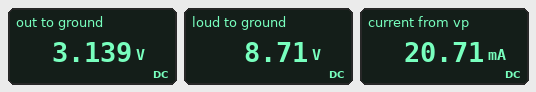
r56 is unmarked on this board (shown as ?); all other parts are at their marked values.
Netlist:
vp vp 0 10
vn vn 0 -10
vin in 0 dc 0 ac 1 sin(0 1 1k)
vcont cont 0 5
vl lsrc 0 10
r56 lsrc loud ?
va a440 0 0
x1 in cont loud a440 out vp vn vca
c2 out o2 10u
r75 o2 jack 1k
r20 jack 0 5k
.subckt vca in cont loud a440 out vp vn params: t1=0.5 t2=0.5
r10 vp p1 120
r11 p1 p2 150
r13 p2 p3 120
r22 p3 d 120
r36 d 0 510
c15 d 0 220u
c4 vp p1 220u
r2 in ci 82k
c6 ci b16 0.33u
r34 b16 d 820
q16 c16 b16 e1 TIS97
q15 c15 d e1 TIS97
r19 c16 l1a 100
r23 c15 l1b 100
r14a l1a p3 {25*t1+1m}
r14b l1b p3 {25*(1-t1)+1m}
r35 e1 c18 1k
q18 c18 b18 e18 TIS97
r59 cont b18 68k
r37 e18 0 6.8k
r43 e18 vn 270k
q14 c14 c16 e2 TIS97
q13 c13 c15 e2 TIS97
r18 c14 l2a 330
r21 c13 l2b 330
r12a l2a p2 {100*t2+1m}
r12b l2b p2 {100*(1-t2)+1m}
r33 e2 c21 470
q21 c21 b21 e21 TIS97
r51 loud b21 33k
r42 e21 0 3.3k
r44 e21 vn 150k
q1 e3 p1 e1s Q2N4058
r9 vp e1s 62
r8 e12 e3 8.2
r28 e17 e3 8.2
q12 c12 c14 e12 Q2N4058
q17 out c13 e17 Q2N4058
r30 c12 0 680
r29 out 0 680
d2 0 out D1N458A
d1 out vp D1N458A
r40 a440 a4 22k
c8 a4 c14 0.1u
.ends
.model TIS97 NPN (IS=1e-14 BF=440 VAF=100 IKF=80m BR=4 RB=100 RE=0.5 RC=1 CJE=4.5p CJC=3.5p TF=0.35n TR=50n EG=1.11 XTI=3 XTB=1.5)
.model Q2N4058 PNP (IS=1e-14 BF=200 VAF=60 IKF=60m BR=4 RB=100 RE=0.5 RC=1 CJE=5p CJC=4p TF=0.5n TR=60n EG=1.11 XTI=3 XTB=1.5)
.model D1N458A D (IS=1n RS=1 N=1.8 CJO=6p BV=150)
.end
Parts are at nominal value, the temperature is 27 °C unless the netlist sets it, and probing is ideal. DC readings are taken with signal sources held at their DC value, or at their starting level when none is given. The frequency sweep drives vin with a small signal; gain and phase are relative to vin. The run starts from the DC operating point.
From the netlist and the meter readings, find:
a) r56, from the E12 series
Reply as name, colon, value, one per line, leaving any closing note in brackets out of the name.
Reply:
r56, from the E12 series: 12 kΩ
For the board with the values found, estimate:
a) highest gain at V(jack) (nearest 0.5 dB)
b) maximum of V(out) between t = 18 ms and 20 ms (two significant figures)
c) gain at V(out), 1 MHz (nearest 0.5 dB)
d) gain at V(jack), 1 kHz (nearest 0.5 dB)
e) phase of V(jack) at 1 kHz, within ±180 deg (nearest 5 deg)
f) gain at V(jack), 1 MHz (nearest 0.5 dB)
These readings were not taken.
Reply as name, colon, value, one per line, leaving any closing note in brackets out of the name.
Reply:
highest gain at V(jack): 4.0 dB
maximum of V(out) between t = 18 ms and 20 ms: 4.9 V
gain at V(out), 1 MHz: 5.0 dB
gain at V(jack), 1 kHz: 4.0 dB
phase of V(jack) at 1 kHz, within ±180 deg: 0 deg
gain at V(jack), 1 MHz: 3.5 dB
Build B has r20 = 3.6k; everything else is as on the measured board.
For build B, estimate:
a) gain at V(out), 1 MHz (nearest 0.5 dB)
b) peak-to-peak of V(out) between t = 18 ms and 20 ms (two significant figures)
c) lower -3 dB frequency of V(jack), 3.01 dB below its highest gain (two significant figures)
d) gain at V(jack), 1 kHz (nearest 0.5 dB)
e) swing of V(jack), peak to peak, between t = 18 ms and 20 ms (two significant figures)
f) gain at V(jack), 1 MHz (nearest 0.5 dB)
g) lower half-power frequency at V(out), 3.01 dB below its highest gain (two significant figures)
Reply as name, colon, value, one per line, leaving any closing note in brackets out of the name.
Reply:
gain at V(out), 1 MHz: 4.5 dB
peak-to-peak of V(out) between t = 18 ms and 20 ms: 3.4 V
lower -3 dB frequency of V(jack), 3.01 dB below its highest gain: 6.9 Hz
gain at V(jack), 1 kHz: 3.0 dB
swing of V(jack), peak to peak, between t = 18 ms and 20 ms: 2.7 V
gain at V(jack), 1 MHz: 2.5 dB
lower half-power frequency at V(out), 3.01 dB below its highest gain: 5.4 Hz
